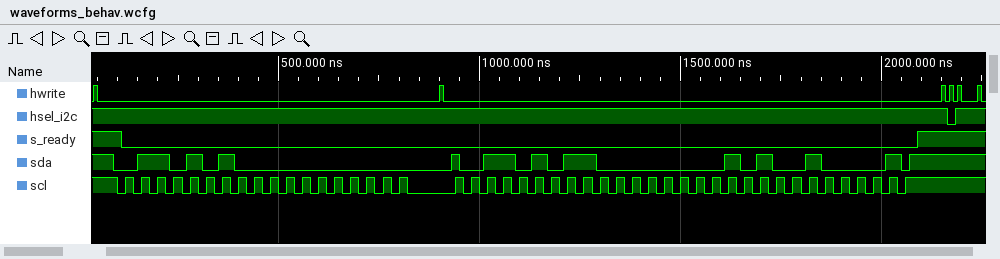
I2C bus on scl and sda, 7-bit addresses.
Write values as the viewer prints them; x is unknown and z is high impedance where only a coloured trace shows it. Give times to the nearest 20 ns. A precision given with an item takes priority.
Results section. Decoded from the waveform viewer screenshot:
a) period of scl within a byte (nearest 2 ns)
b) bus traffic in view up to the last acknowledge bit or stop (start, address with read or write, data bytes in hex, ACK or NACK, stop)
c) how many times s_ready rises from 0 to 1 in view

40 ns
start, address 35 write ACK, 00 ACK, repeated start, address 35 read ACK, 01 ACK, 90 NACK, stop
1
